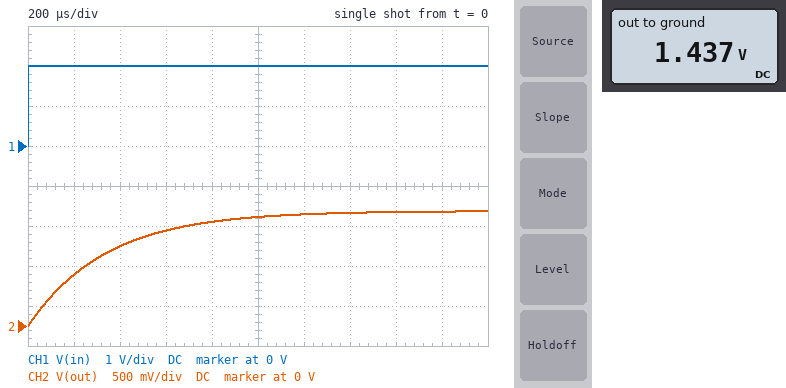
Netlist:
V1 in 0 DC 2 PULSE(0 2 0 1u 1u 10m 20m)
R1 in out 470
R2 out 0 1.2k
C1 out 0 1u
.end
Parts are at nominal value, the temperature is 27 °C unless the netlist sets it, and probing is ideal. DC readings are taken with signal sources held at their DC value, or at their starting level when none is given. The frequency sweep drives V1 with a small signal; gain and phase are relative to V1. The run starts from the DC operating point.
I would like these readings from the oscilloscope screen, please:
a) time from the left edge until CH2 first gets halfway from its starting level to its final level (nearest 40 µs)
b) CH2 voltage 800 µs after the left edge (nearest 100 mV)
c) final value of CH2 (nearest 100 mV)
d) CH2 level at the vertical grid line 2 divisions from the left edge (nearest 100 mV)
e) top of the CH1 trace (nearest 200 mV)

240 µs
1.3 V
1.4 V
1.0 V
2.0 V
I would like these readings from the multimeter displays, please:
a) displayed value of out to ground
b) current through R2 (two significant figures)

1.437 V
1.2 mA
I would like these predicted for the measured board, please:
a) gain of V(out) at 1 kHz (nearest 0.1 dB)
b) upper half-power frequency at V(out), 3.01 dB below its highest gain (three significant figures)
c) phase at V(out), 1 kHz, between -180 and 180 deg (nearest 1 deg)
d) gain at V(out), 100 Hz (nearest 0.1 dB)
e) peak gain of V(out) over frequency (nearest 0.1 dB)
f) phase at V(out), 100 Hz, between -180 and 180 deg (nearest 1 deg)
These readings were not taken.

-10.3 dB
471 Hz
-65 deg
-3.1 dB
-2.9 dB
-12 deg
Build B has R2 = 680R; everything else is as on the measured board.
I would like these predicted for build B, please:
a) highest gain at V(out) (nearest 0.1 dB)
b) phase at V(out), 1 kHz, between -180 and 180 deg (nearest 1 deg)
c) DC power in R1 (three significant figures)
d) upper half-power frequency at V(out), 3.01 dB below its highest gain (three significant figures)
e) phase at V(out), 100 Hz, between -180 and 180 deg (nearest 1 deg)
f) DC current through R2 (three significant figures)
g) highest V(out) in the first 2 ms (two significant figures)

-4.6 dB
-60 deg
1.42 mW
573 Hz
-10 deg
1.74 mA
1.2 V
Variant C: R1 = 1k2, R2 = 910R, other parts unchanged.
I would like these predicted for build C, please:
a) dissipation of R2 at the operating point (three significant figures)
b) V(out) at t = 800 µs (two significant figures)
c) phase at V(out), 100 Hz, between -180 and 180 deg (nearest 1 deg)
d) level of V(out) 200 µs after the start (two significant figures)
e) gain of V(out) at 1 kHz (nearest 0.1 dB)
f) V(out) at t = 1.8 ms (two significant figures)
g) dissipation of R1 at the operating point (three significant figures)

818 µW
680 mV
-18 deg
280 mV
-17.9 dB
840 mV
1.08 mW
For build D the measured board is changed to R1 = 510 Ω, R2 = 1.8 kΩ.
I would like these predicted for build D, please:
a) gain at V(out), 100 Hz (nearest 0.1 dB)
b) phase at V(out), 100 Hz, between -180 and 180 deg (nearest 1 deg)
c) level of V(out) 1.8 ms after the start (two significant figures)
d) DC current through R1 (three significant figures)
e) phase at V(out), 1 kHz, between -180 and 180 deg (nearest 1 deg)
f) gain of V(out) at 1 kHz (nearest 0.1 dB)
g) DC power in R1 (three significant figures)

-2.4 dB
-14 deg
1.5 V
866 µA
-68 deg
-10.8 dB
382 µW
